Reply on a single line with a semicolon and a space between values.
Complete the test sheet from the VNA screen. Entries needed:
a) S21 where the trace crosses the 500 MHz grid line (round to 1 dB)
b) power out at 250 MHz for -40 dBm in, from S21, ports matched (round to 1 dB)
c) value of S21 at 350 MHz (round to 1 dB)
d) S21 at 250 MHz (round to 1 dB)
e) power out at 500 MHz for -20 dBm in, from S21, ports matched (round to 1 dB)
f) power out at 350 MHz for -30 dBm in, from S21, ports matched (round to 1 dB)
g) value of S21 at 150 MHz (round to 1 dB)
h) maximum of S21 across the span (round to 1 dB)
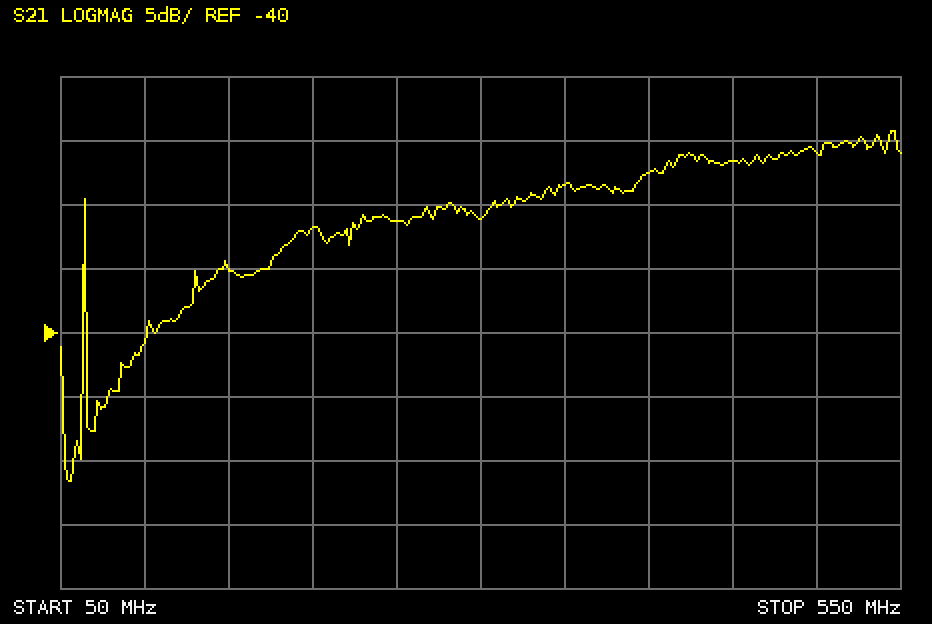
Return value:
-26 dB; -71 dBm; -28 dB; -31 dB; -46 dBm; -58 dBm; -35 dB; -24 dB
